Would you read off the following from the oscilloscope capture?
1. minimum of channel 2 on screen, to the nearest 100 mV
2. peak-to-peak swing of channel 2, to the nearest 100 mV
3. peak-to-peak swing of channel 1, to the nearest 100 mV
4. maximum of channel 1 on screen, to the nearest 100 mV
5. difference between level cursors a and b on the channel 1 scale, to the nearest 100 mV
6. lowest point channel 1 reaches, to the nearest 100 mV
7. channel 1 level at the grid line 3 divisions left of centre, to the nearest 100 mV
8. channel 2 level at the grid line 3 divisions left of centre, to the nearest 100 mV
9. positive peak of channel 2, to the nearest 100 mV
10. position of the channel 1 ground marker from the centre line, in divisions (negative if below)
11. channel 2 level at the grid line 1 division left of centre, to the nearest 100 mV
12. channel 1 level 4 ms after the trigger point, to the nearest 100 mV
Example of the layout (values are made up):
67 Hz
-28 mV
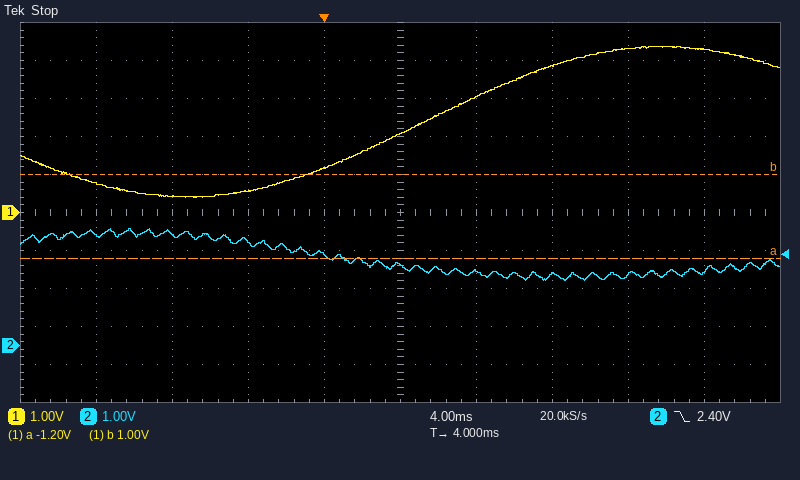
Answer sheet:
1.7 V
1.4 V
4.0 V
4.4 V
2.2 V
400 mV
400 mV
2.9 V
3.1 V
0.0 div
2.4 V
2.1 V
